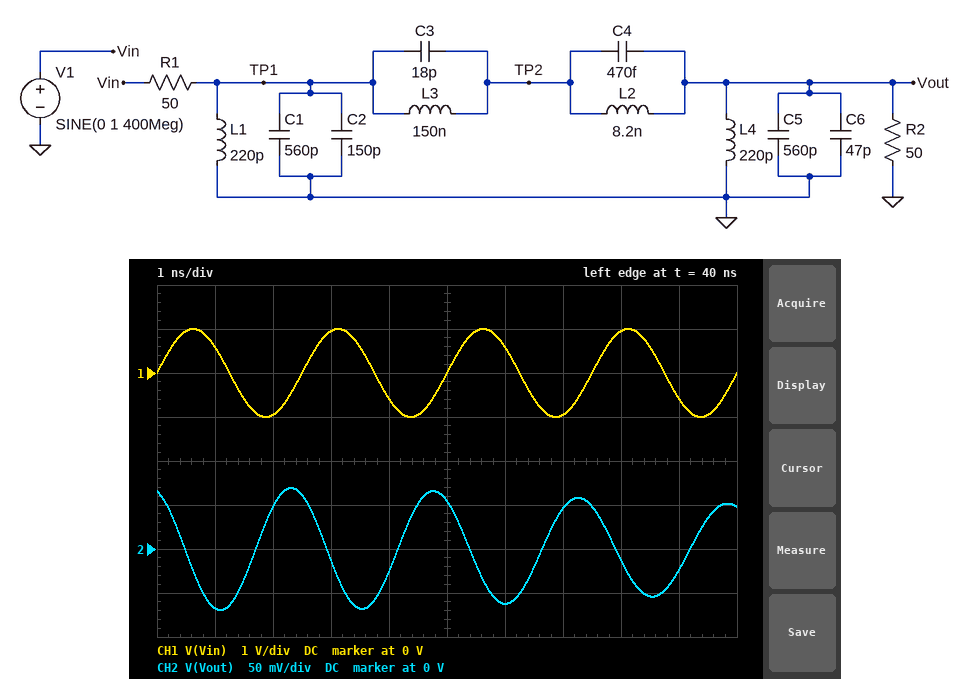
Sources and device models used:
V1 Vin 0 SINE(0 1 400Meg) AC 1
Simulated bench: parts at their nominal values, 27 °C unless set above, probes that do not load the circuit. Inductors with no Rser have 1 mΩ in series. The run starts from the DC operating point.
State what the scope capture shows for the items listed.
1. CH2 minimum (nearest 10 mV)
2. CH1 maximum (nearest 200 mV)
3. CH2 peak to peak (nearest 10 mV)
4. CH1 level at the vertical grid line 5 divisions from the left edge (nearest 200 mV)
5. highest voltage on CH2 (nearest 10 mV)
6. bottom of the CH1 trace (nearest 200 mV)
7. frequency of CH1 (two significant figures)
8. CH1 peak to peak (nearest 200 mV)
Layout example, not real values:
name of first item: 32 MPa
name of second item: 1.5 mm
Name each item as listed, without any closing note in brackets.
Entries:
CH2 minimum: -70 mV
CH1 maximum: 1.0 V
CH2 peak to peak: 140 mV
CH1 level at the vertical grid line 5 divisions from the left edge: 0 V
highest voltage on CH2: 70 mV
bottom of the CH1 trace: -1.0 V
frequency of CH1: 400 MHz
CH1 peak to peak: 2.0 V
